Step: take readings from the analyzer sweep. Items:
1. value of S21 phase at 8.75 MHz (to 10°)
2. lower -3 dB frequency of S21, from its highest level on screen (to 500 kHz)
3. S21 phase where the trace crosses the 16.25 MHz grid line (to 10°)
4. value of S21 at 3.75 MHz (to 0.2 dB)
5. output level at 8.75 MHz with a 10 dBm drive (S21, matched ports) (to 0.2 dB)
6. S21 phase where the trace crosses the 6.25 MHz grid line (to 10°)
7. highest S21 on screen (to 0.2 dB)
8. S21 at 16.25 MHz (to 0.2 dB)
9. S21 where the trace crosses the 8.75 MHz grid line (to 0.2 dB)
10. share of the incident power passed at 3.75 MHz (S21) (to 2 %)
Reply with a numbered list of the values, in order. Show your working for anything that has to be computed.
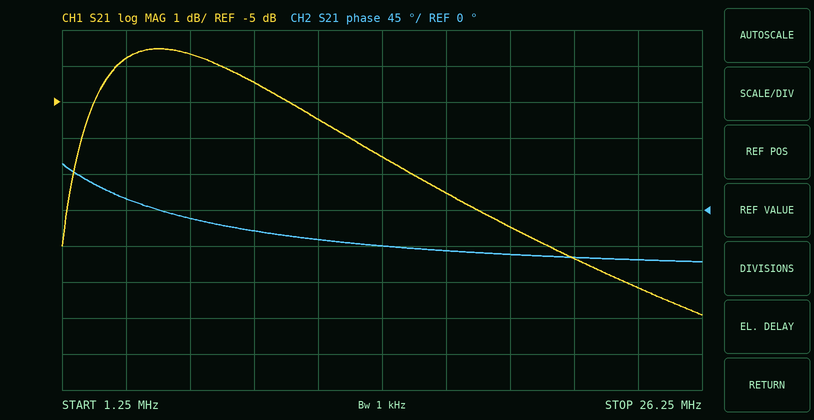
1. -30°
2. 2.0 MHz
3. -50°
4. -3.8 dB
5. 10 dBm + (-4.4 dB) = 5.6 dBm
6. -10°
7. -3.6 dB
8. -7.6 dB
9. -4.4 dB
10. 10^(-3.8/10) ≈ 42 %
